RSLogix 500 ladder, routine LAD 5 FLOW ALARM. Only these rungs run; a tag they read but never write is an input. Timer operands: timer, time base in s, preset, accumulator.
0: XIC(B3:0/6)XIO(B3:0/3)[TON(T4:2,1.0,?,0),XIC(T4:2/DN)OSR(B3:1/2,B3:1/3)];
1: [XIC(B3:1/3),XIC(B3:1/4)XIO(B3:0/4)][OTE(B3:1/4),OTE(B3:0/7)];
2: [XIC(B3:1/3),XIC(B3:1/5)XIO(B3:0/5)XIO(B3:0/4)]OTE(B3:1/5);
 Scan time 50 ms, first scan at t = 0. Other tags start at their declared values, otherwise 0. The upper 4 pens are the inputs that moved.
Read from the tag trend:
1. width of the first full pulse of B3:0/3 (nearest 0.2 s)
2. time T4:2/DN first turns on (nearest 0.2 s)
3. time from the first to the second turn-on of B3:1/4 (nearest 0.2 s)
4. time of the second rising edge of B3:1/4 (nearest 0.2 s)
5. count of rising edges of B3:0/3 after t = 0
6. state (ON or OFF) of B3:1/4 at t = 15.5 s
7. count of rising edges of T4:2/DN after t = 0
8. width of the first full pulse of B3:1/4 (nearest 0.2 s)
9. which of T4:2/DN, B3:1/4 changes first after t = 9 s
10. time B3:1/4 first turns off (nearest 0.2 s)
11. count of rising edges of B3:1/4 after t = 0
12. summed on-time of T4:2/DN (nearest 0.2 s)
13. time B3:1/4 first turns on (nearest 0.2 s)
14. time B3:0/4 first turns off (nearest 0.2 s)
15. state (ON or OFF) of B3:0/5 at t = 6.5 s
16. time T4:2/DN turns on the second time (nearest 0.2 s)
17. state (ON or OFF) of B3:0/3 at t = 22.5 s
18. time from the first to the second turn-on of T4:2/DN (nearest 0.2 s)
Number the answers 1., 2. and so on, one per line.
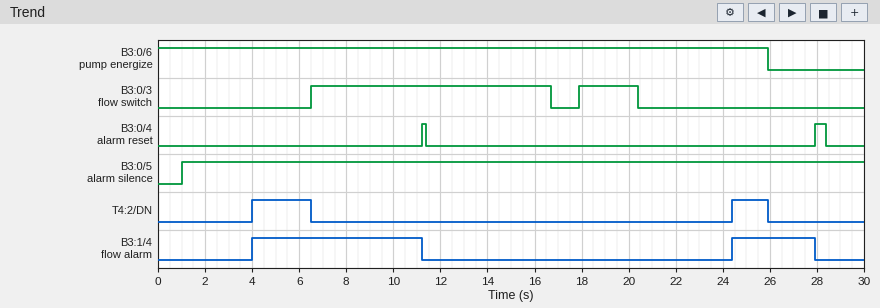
1. 10.2 s
2. 4.0 s
3. 20.4 s
4. 24.4 s
5. 2
6. OFF
7. 2
8. 7.2 s
9. B3:1/4
10. 11.2 s
11. 2
12. 4.0 s
13. 4.0 s
14. 11.4 s
15. ON
16. 24.4 s
17. OFF
18. 20.4 s
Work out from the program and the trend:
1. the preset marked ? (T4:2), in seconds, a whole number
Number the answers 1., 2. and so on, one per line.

1. 4 s
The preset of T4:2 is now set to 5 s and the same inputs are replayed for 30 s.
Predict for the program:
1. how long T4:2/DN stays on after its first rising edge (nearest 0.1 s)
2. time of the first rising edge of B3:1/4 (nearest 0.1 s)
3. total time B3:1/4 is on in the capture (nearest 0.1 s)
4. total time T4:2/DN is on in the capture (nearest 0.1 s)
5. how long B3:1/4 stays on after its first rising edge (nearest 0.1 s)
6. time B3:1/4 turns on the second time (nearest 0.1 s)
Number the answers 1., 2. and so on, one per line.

1. 1.5 s
2. 5.0 s
3. 8.7 s
4. 2.0 s
5. 6.2 s
6. 25.4 s
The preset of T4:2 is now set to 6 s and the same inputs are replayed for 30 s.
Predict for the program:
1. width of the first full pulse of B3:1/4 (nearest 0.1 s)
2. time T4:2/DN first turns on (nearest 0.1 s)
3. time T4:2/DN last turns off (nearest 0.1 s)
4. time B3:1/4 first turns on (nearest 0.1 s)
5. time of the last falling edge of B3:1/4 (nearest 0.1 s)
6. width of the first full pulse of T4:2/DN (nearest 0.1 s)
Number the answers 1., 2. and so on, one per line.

1. 5.2 s
2. 6.0 s
3. 6.5 s
4. 6.0 s
5. 11.2 s
6. 0.5 s
